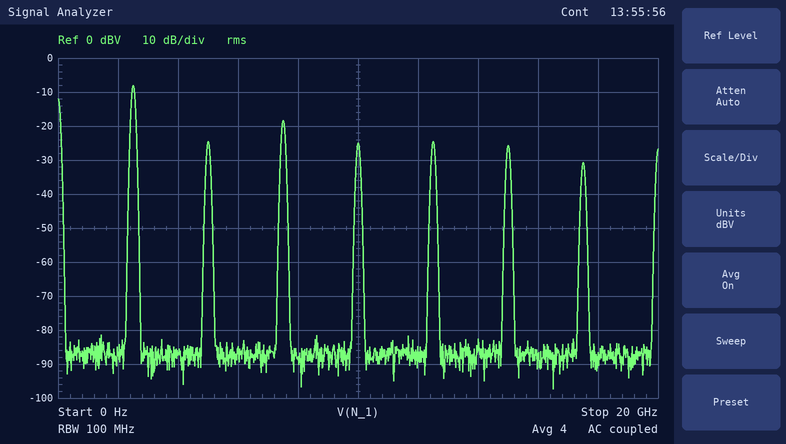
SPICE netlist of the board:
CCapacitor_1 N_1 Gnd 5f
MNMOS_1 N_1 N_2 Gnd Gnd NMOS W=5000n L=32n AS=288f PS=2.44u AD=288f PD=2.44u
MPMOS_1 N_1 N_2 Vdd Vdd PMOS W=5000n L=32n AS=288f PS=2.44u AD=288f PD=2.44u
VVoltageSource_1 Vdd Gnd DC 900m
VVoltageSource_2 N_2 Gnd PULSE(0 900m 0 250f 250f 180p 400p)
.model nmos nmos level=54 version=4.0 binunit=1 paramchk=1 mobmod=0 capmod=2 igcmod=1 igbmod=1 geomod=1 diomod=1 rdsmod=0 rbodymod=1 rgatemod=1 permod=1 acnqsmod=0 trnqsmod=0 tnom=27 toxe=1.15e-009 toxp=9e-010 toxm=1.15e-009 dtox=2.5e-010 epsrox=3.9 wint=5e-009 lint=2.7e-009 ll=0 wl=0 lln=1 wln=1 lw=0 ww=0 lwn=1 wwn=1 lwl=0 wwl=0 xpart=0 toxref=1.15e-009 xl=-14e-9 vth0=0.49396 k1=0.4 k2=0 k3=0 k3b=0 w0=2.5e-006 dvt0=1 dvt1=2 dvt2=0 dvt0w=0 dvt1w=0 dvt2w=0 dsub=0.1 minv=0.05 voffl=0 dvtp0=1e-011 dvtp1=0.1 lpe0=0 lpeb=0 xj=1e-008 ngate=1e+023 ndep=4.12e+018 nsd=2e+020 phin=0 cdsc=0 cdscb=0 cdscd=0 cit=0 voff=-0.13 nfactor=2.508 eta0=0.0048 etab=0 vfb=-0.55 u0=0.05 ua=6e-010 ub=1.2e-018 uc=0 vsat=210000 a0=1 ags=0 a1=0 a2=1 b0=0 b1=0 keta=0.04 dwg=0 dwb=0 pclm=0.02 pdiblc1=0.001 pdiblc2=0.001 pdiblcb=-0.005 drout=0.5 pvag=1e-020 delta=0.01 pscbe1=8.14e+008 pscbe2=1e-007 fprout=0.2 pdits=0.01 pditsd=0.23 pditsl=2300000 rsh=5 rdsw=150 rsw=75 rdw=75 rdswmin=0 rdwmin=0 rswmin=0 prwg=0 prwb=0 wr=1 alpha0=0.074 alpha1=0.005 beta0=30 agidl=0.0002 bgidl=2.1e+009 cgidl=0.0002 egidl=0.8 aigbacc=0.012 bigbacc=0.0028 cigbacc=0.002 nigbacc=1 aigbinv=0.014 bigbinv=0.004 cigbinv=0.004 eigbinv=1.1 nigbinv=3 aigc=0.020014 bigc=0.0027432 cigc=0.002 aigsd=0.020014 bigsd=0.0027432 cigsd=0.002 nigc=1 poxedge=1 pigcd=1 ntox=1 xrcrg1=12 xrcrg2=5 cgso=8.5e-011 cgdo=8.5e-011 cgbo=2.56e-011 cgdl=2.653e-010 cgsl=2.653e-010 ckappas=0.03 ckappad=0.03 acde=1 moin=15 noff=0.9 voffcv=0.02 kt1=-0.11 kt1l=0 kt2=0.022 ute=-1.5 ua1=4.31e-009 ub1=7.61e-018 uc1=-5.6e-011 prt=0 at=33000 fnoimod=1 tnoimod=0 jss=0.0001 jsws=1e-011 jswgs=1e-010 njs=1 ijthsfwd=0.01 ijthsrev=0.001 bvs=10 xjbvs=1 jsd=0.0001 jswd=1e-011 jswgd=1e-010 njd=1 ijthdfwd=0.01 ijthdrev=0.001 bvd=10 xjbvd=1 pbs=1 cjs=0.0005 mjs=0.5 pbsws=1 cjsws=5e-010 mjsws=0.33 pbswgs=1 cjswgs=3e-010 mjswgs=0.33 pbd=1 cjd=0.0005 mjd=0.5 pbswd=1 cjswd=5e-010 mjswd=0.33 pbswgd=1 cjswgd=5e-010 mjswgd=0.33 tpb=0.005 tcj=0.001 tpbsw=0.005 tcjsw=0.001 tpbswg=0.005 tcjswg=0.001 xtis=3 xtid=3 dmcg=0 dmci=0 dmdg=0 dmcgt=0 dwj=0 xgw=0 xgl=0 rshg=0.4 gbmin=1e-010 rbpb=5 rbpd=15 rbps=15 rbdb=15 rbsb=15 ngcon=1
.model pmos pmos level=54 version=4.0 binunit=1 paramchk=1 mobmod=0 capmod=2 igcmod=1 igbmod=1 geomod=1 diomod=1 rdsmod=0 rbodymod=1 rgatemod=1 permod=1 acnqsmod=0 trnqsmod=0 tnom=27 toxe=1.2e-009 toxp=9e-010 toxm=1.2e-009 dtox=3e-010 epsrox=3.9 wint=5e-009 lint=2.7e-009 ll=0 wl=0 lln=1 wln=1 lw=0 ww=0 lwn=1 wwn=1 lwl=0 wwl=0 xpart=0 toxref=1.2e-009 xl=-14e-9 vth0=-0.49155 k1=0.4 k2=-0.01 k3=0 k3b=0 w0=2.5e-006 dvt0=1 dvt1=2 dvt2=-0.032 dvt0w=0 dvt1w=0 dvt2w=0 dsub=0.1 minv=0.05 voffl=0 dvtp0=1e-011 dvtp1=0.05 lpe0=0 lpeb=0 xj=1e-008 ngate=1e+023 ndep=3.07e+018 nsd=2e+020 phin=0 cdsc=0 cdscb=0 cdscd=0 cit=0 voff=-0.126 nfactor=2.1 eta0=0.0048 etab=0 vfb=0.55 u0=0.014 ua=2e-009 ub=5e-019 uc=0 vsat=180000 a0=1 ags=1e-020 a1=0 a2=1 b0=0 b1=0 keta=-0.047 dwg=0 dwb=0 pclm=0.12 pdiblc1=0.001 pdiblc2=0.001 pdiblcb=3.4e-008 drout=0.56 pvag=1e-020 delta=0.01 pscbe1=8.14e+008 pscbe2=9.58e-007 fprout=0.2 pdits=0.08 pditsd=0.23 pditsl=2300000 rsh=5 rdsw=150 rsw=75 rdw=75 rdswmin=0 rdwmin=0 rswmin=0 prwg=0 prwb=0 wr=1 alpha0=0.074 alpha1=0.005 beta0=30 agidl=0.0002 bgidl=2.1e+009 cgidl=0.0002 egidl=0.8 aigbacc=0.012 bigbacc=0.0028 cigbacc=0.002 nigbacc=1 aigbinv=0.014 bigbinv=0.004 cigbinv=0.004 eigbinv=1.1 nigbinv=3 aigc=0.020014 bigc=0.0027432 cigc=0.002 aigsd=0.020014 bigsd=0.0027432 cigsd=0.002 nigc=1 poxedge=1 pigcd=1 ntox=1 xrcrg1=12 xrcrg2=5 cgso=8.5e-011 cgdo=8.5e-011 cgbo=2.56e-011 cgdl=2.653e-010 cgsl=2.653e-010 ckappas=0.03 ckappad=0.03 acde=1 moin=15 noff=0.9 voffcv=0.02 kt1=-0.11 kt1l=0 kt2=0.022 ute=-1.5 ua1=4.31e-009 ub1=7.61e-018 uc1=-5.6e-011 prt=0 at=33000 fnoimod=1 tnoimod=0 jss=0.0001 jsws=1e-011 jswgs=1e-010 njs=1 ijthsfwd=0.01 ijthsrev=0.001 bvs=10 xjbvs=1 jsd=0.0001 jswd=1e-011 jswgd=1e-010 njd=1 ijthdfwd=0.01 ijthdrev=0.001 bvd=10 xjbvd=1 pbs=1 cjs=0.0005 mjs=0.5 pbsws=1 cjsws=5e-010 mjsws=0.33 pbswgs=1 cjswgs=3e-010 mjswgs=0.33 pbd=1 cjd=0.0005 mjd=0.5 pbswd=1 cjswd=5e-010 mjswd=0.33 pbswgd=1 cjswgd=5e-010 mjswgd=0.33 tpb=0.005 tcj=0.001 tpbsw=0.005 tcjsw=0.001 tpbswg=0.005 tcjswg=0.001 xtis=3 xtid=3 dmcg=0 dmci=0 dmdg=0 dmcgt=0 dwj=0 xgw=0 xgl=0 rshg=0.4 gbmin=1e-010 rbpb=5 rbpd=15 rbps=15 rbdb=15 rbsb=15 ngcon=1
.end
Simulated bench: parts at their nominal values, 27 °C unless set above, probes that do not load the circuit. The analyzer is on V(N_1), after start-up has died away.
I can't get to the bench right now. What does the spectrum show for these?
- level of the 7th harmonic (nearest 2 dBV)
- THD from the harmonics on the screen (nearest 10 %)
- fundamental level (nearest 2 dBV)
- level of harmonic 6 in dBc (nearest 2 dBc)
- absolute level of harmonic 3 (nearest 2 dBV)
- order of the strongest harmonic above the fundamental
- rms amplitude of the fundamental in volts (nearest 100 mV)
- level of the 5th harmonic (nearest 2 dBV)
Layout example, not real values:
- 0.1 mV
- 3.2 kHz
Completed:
- -30 dBV
- 40 %
- -8 dBV
- -18 dBc
- -18 dBV
- 3
- 400 mV
- -24 dBV
